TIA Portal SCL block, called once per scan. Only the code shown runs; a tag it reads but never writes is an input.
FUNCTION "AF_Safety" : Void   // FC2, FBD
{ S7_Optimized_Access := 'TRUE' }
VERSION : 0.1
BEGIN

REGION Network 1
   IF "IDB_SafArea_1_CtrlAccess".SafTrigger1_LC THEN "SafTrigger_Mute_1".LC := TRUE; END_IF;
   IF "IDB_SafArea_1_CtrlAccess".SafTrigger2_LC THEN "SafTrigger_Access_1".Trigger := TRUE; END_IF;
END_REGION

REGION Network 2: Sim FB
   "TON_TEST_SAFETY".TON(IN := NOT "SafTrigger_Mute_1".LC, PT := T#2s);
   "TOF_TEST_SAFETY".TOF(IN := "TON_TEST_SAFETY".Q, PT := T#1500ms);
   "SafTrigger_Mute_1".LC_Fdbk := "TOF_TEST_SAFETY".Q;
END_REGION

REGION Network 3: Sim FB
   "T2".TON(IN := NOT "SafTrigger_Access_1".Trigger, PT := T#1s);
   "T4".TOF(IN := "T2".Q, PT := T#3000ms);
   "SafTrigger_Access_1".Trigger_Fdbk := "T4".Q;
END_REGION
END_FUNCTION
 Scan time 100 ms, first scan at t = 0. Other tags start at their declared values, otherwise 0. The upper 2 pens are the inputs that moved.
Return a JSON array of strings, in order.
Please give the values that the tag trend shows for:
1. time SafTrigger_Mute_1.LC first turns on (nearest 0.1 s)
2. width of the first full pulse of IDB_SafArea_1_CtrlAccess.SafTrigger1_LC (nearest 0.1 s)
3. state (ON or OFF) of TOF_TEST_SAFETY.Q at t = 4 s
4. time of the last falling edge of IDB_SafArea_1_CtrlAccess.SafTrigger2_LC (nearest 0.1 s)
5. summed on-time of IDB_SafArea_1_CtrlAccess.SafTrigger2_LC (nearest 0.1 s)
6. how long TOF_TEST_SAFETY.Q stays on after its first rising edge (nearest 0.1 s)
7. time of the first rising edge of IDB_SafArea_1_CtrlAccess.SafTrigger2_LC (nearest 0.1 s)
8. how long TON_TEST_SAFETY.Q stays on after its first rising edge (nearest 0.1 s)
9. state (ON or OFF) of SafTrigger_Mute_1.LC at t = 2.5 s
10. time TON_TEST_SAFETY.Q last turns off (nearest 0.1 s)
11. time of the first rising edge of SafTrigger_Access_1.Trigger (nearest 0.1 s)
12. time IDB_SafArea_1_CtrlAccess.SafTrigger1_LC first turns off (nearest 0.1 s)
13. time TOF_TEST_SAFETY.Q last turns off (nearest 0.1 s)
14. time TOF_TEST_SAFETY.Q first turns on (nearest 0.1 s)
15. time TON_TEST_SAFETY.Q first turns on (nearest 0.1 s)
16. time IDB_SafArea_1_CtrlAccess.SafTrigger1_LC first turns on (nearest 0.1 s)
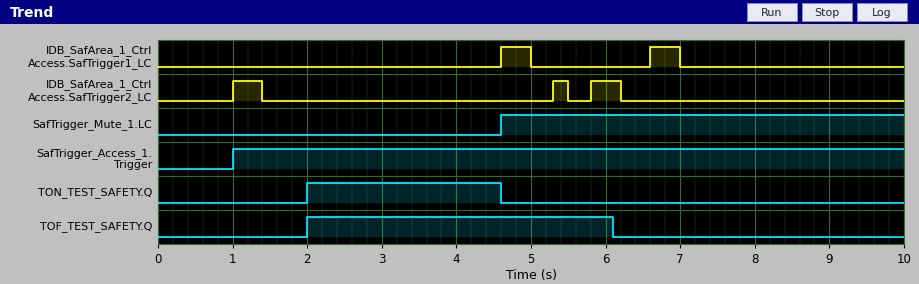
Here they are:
["4.6 s", "0.4 s", "ON", "6.2 s", "1.0 s", "4.1 s", "1.0 s", "2.6 s", "OFF", "4.6 s", "1.0 s", "5.0 s", "6.1 s", "2.0 s", "2.0 s", "4.6 s"]
